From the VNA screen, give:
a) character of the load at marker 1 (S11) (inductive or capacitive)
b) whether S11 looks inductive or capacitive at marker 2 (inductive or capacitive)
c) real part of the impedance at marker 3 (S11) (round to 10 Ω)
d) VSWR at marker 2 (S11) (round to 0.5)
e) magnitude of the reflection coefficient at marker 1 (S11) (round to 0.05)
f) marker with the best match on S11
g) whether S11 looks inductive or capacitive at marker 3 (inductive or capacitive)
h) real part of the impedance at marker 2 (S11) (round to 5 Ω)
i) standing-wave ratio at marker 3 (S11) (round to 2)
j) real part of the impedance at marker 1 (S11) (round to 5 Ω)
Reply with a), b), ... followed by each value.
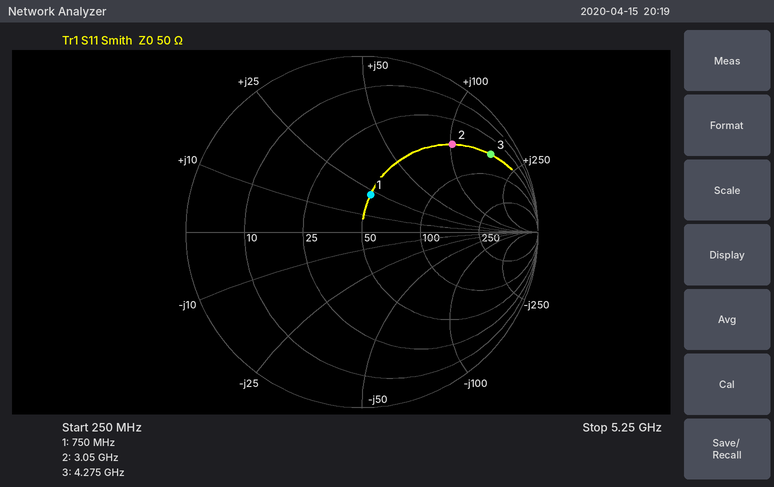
a) inductive
b) inductive
c) 50 Ω
d) 6.0
e) 0.20
f) marker 1
g) inductive
h) 50 Ω
i) 12
j) 50 Ω
